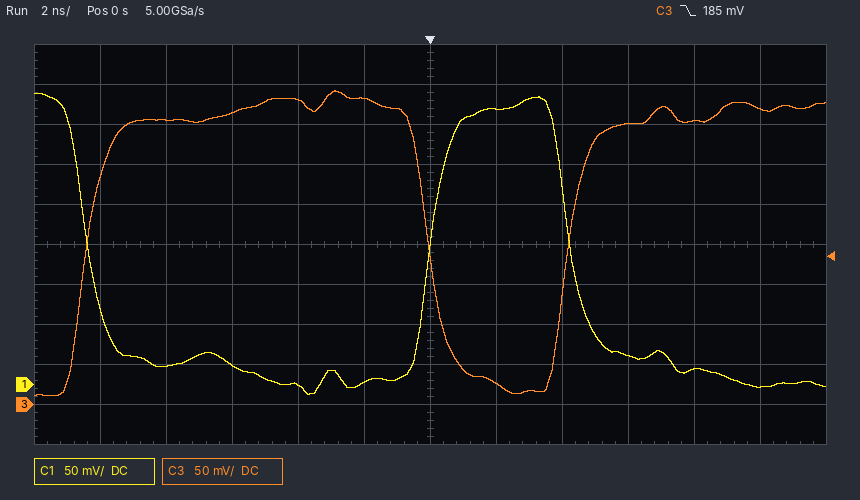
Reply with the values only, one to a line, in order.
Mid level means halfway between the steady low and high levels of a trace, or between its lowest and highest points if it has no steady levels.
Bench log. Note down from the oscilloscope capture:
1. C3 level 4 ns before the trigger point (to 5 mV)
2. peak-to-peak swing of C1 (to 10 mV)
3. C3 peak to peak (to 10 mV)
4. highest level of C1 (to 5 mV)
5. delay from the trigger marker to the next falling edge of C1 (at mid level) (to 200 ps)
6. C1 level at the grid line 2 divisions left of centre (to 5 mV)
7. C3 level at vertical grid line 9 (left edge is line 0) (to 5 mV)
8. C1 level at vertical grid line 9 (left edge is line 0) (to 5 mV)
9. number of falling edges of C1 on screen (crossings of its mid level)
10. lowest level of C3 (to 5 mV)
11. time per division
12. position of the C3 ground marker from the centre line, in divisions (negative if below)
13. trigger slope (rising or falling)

380 mV
380 mV
380 mV
365 mV
4.2 ns
0 mV
350 mV
35 mV
2
10 mV
2 ns
-4.0 div
falling
